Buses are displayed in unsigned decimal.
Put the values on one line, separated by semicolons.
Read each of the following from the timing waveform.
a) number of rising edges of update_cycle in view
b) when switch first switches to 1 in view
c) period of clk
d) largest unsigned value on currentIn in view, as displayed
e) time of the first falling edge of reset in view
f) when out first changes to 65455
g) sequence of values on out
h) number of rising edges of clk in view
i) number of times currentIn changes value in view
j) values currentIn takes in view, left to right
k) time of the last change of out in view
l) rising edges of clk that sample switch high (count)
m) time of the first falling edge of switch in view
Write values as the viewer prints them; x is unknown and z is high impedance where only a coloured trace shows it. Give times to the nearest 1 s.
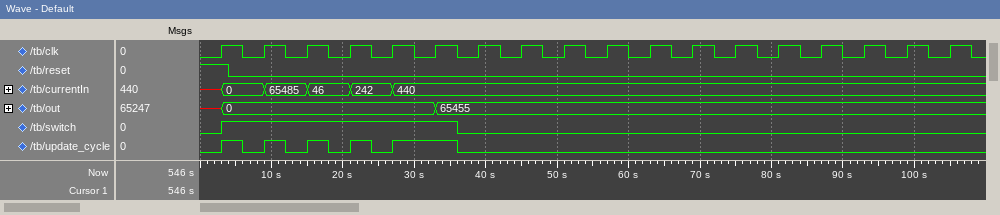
5; 3 s; 6 s; 65485; 4 s; 33 s; x, 0, 65455; 18; 5; x, 0, 65485, 46, 242, 440; 33 s; 5; 36 s
